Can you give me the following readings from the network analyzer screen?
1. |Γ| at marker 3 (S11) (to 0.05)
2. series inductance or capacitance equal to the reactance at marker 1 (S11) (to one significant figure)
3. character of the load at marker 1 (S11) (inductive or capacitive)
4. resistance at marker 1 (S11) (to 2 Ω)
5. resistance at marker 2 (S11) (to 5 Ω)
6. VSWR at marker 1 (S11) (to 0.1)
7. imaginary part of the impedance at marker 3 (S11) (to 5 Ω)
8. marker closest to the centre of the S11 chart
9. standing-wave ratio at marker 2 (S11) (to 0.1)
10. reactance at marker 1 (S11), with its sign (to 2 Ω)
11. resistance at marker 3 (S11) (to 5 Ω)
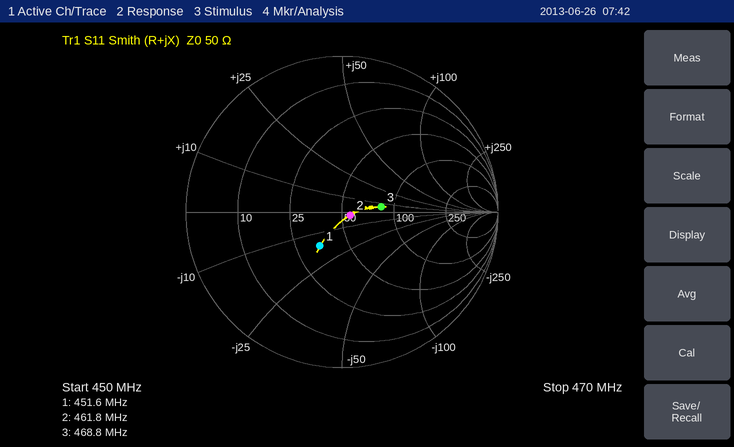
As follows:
0.25
20 pF
capacitive
34 Ω
55 Ω
1.7
+5 Ω
marker 2
1.1
-16 Ω
85 Ω
